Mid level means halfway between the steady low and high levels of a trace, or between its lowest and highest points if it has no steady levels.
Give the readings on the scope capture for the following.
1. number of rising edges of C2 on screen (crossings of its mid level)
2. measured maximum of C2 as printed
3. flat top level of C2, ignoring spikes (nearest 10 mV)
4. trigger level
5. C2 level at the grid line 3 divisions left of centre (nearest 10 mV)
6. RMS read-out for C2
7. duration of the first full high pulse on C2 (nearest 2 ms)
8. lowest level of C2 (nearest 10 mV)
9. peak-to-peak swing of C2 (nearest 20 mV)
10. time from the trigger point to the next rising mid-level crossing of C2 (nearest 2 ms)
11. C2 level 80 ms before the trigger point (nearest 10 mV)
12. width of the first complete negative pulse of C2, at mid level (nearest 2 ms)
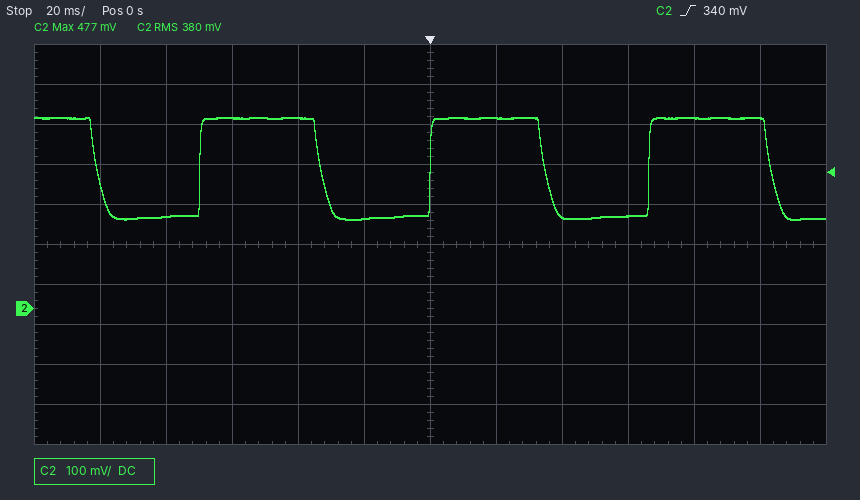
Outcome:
3
477 mV
480 mV
340 mV
480 mV
380 mV
36 ms
220 mV
260 mV
66 ms
230 mV
32 ms
